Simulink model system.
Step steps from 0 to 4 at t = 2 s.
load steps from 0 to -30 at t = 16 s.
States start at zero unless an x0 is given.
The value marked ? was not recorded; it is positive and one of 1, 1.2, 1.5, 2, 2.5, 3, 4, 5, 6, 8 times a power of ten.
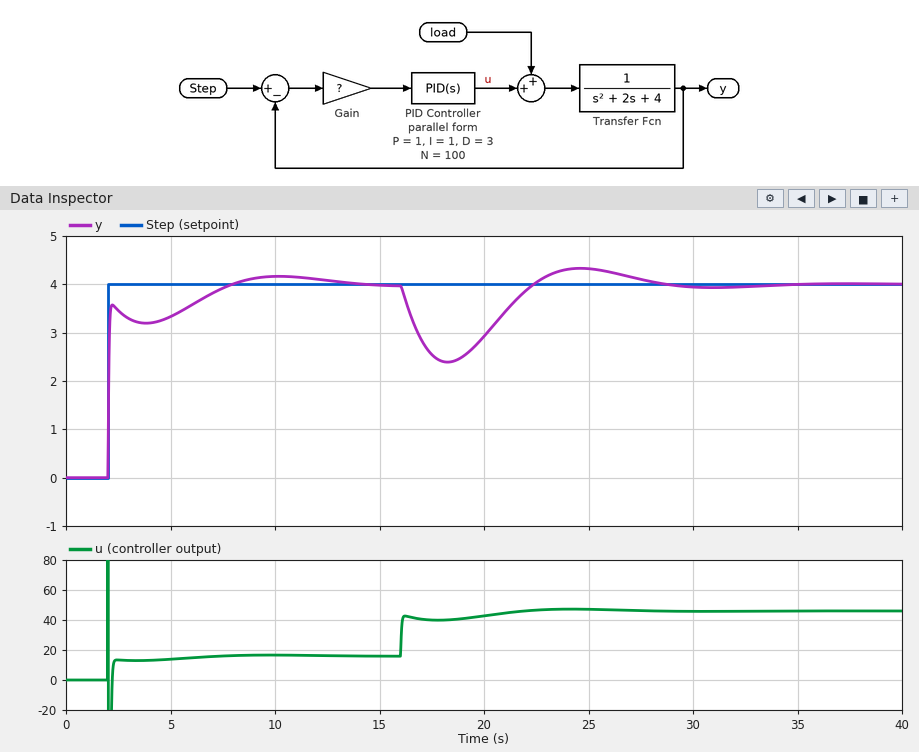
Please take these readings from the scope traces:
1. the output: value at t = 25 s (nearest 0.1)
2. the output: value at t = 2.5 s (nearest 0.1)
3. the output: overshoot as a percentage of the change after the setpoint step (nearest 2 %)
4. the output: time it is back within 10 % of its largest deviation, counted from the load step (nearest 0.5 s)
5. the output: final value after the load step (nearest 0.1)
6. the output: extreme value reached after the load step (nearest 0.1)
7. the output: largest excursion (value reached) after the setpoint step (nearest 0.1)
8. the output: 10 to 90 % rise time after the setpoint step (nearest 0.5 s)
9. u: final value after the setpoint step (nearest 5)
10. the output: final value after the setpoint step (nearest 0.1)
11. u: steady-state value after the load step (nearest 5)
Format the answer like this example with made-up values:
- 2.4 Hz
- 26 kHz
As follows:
- 4.3
- 3.5
- 4 %
- 11.0 s
- 4.0
- 2.4
- 4.2
- 4.0 s
- 15
- 4.0
- 45
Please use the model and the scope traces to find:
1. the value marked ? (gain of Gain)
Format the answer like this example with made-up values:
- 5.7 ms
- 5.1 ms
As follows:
- 6
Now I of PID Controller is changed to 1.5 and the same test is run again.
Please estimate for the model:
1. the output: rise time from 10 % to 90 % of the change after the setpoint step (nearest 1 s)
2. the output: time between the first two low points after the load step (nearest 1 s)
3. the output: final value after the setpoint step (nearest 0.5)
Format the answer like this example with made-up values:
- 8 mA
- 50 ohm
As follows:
- 3 s
- 10 s
- 4.0
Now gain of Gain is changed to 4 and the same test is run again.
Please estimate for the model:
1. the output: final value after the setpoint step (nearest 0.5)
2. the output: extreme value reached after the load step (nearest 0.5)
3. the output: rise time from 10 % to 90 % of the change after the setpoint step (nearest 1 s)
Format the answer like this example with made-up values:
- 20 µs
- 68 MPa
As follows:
- 4.0
- 2.0
- 5 s
